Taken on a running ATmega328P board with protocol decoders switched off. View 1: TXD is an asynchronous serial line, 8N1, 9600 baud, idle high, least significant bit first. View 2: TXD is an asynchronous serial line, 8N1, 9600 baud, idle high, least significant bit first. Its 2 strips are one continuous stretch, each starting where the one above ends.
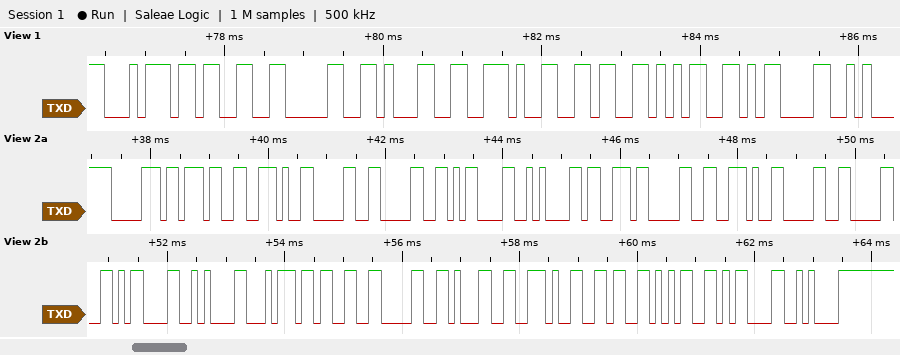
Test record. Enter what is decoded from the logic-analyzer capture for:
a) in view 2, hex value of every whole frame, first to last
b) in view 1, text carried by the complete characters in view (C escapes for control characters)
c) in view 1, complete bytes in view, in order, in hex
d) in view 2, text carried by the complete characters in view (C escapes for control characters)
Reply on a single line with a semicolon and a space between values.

70 37 2E 30 30 0D 0A 73 30 2E 30 30 0D 0A 74 33 30 31 2E 36 35 0D 0A; "t301.65\r"; 74 33 30 31 2E 36 35 0D; "p7.00\r\ns0.00\r\nt301.65\r\n"
